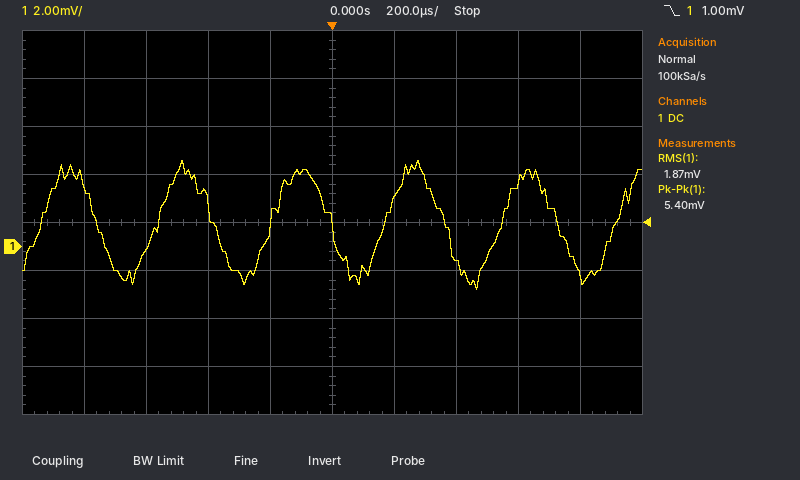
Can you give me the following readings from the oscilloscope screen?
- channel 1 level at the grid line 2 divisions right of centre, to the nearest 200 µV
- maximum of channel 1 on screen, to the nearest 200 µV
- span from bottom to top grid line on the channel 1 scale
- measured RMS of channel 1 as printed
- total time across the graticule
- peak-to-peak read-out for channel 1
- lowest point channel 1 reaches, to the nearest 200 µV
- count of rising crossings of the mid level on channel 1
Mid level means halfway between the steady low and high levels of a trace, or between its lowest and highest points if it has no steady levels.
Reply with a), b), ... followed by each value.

a) -600 µV
b) 3.6 mV
c) 16 mV
d) 1.87 mV
e) 2 ms
f) 5.40 mV
g) -1.8 mV
h) 6
